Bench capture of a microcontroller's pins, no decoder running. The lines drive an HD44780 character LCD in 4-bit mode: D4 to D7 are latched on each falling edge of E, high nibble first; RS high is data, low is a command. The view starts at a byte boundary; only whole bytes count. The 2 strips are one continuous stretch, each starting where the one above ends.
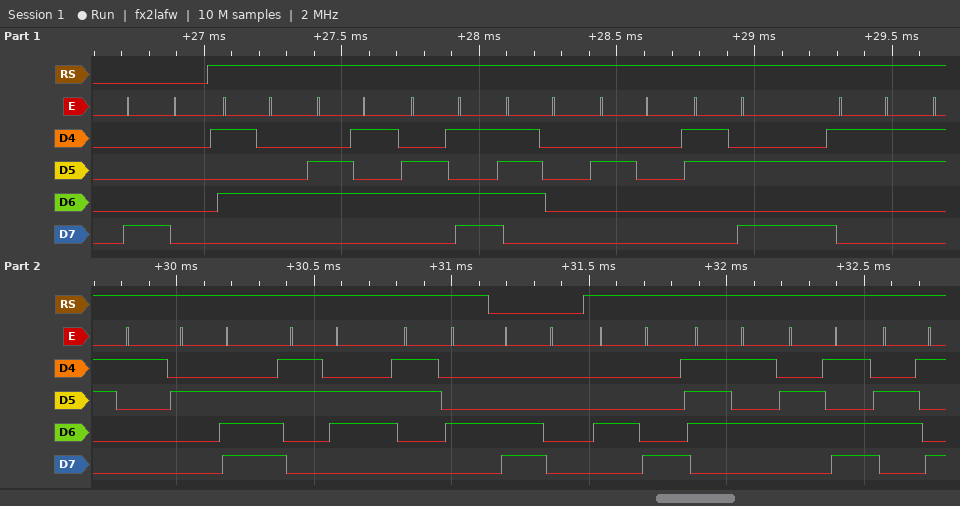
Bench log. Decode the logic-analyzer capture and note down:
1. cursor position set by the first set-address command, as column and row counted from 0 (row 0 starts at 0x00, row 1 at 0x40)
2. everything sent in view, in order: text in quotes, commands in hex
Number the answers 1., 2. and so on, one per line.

1. column 0, row 0
2. 0x80 "Temp :31.64" 0xC0 "Humi"
